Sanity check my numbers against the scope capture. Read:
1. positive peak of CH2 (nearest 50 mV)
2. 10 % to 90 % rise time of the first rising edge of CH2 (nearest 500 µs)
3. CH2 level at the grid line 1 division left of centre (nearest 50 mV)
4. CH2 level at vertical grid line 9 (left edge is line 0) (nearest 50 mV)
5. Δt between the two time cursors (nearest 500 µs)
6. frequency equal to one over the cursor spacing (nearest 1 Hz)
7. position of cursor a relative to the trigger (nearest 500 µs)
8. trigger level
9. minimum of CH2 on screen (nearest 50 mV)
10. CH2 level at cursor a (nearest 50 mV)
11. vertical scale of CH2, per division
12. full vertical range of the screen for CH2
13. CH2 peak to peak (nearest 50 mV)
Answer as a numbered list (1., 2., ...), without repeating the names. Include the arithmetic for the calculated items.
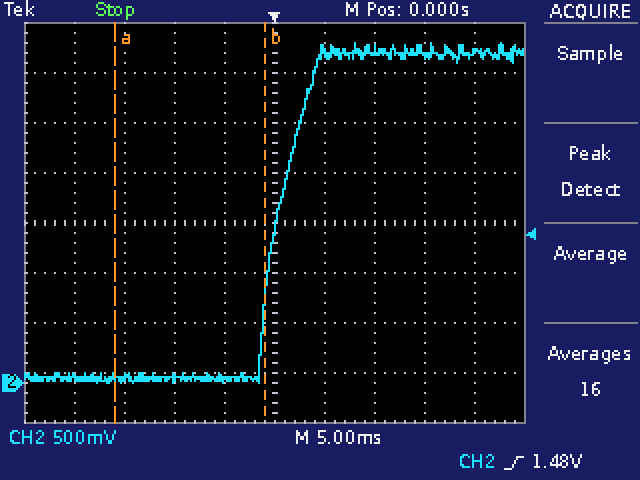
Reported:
1. 3.40 V
2. 5.0 ms
3. 50 mV
4. 3.30 V
5. 15.0 ms
6. 1 / 15.0 ms ≈ 67 Hz
7. -16.0 ms
8. 1.48 V
9. 0 mV
10. 50 mV
11. 500 mV
12. 4 V
13. 3.40 V − (0 mV) = 3.40 V
